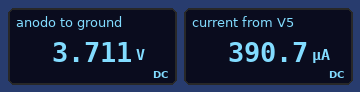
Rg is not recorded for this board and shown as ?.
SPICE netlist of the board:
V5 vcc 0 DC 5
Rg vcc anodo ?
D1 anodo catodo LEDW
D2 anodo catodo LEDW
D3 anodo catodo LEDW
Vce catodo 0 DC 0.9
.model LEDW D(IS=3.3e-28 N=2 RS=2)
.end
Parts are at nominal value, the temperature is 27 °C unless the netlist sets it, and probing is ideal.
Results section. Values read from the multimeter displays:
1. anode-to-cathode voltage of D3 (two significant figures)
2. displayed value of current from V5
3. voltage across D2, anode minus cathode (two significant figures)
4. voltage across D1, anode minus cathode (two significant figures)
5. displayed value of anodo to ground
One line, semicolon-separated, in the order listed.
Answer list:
2.8 V; 390.7 µA; 2.8 V; 2.8 V; 3.711 V
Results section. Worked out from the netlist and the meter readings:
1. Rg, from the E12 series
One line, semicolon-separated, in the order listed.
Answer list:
3.3 kΩ
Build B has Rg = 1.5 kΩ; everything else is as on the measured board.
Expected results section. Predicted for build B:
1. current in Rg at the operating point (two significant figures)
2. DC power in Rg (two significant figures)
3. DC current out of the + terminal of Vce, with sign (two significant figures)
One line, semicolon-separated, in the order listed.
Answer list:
830 µA; 1.0 mW; -830 µA
